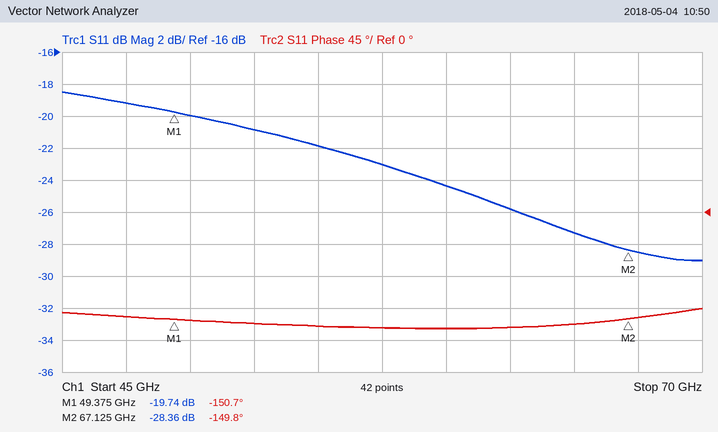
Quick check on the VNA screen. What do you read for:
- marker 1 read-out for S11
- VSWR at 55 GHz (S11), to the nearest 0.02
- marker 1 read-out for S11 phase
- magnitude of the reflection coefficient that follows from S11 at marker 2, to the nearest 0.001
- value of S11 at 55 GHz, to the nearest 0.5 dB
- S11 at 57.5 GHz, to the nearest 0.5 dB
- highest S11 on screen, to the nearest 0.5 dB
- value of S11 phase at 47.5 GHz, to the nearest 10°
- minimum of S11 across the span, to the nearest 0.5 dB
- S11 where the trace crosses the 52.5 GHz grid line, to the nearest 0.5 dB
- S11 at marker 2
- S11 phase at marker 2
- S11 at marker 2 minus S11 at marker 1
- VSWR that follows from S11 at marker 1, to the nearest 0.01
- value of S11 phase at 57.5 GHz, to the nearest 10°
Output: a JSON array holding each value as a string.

["-19.74 dB", "1.18", "-150.7°", "0.038", "-22.0 dB", "-23.0 dB", "-18.5 dB", "-150°", "-29.0 dB", "-21.0 dB", "-28.36 dB", "-149.8°", "-8.62 dB", "1.23", "-160°"]
